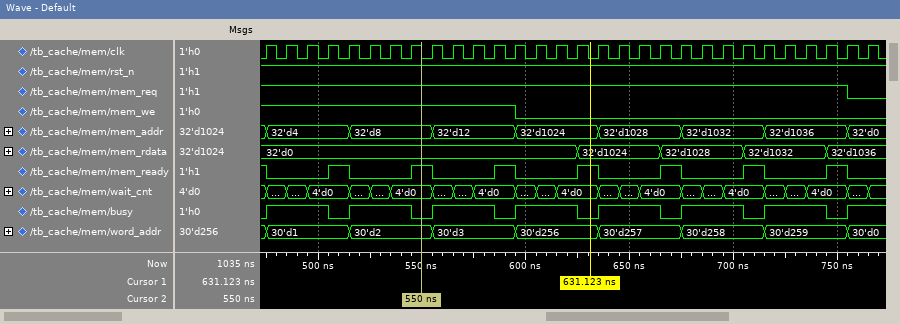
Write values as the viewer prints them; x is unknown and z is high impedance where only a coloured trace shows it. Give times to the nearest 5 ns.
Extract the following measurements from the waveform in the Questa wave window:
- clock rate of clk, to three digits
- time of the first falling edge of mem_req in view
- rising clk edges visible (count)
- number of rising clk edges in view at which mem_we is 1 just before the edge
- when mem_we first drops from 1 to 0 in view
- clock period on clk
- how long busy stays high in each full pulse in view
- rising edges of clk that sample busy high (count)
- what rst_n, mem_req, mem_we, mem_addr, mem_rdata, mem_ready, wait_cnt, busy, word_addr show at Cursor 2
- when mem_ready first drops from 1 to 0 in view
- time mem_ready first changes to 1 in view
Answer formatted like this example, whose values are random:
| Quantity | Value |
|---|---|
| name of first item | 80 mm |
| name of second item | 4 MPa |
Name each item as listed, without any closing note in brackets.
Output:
| Quantity | Value |
|---|---|
| clock rate of clk, to three digits | 100 MHz |
| time of the first falling edge of mem_req in view | 755 ns |
| rising clk edges visible | 30 |
| number of rising clk edges in view at which mem_we is 1 just before the edge | 13 |
| when mem_we first drops from 1 to 0 in view | 595 ns |
| clock period on clk | 10 ns |
| how long busy stays high in each full pulse in view | 30 ns, 30 ns, 30 ns, 30 ns, 30 ns, 30 ns, 30 ns |
| rising edges of clk that sample busy high | 22 |
| what rst_n, mem_req, mem_we, mem_addr, mem_rdata, mem_ready, wait_cnt, busy, word_addr show at Cursor 2 | rst_n=1, mem_req=1, mem_we=1, mem_addr=32'd8, mem_rdata=32'd0, mem_ready=1, wait_cnt=4'd0, busy=0, word_addr=30'd2 |
| when mem_ready first drops from 1 to 0 in view | 475 ns |
| time mem_ready first changes to 1 in view | 505 ns |
